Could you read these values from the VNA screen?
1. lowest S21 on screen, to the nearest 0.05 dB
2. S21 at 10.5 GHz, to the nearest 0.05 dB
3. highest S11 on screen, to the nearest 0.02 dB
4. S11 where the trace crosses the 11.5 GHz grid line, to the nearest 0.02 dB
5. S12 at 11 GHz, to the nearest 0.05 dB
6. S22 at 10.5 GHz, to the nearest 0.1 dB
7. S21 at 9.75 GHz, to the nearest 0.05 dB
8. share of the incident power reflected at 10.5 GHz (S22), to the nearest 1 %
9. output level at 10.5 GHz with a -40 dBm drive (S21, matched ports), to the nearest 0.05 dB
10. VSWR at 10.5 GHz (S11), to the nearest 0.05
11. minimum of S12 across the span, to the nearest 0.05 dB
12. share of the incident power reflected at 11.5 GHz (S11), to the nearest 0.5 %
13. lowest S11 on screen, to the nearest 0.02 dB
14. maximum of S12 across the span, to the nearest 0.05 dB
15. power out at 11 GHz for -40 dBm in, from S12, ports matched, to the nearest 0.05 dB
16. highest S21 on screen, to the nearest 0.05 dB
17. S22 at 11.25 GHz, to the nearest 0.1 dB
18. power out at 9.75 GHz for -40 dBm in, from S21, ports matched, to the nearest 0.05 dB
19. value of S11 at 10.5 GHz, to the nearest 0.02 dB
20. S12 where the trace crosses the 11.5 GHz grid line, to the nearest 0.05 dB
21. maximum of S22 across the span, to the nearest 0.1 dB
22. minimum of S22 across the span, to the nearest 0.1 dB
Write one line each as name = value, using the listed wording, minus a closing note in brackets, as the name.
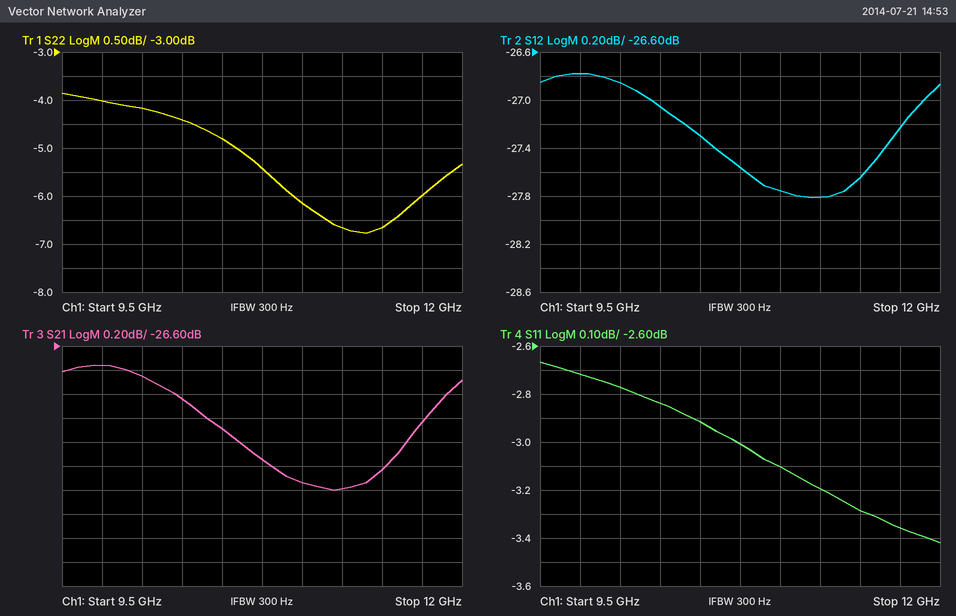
lowest S21 on screen, to the nearest 0.05 dB = -27.80 dB
S21 at 10.5 GHz, to the nearest 0.05 dB = -27.30 dB
highest S11 on screen, to the nearest 0.02 dB = -2.66 dB
S11 where the trace crosses the 11.5 GHz grid line, to the nearest 0.02 dB = -3.28 dB
S12 at 11 GHz, to the nearest 0.05 dB = -27.75 dB
S22 at 10.5 GHz, to the nearest 0.1 dB = -4.8 dB
S21 at 9.75 GHz, to the nearest 0.05 dB = -26.75 dB
share of the incident power reflected at 10.5 GHz (S22), to the nearest 1 % = 33 %
output level at 10.5 GHz with a -40 dBm drive (S21, matched ports), to the nearest 0.05 dB = -67.30 dBm
VSWR at 10.5 GHz (S11), to the nearest 0.05 = 6.00
minimum of S12 across the span, to the nearest 0.05 dB = -27.80 dB
share of the incident power reflected at 11.5 GHz (S11), to the nearest 0.5 % = 47.0 %
lowest S11 on screen, to the nearest 0.02 dB = -3.42 dB
maximum of S12 across the span, to the nearest 0.05 dB = -26.80 dB
power out at 11 GHz for -40 dBm in, from S12, ports matched, to the nearest 0.05 dB = -67.75 dBm
highest S21 on screen, to the nearest 0.05 dB = -26.75 dB
S22 at 11.25 GHz, to the nearest 0.1 dB = -6.7 dB
power out at 9.75 GHz for -40 dBm in, from S21, ports matched, to the nearest 0.05 dB = -66.75 dBm
value of S11 at 10.5 GHz, to the nearest 0.02 dB = -2.92 dB
S12 where the trace crosses the 11.5 GHz grid line, to the nearest 0.05 dB = -27.65 dB
maximum of S22 across the span, to the nearest 0.1 dB = -3.9 dB
minimum of S22 across the span, to the nearest 0.1 dB = -6.8 dB
